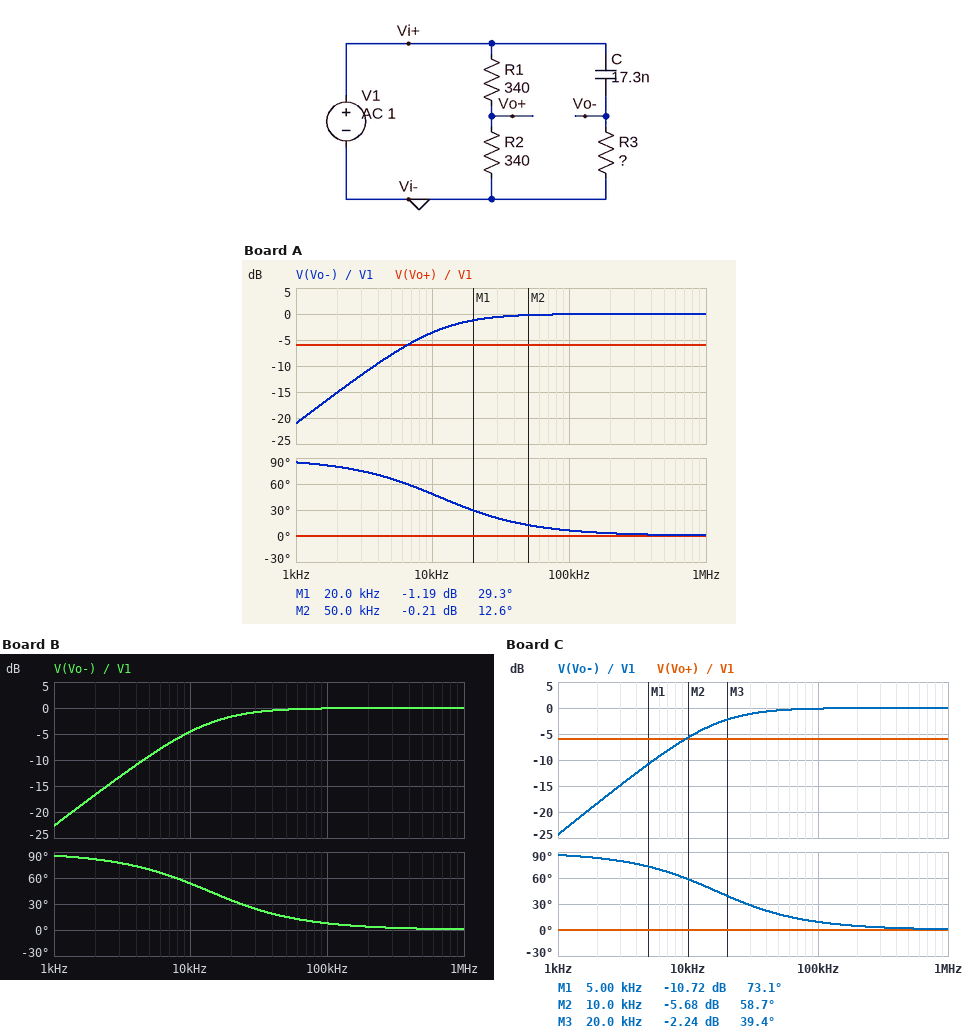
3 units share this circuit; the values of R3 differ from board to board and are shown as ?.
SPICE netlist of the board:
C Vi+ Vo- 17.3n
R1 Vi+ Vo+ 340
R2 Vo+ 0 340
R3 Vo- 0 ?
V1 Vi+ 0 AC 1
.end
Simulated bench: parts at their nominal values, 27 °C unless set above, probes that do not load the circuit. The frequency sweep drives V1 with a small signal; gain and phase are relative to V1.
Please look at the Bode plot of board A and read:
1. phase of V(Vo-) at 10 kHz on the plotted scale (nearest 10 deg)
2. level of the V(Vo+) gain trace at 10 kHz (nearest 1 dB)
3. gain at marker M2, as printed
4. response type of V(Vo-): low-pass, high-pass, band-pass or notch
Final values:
50 deg
-6 dB
-0.21 dB
high-pass
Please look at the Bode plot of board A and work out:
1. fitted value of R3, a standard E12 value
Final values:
820 Ω
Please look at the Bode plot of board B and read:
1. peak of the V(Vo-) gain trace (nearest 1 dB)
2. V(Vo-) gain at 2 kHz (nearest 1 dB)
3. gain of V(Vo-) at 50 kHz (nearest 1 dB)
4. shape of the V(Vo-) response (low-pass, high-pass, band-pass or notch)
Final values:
0 dB
-17 dB
0 dB
high-pass
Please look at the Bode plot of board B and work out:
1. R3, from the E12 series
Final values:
680 Ω
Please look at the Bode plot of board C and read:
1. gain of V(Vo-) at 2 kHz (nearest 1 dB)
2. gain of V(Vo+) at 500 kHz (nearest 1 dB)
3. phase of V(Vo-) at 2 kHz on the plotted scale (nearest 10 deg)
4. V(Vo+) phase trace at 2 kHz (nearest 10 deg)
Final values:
-18 dB
-6 dB
80 deg
0 deg
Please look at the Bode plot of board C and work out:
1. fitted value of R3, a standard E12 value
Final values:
560 Ω
